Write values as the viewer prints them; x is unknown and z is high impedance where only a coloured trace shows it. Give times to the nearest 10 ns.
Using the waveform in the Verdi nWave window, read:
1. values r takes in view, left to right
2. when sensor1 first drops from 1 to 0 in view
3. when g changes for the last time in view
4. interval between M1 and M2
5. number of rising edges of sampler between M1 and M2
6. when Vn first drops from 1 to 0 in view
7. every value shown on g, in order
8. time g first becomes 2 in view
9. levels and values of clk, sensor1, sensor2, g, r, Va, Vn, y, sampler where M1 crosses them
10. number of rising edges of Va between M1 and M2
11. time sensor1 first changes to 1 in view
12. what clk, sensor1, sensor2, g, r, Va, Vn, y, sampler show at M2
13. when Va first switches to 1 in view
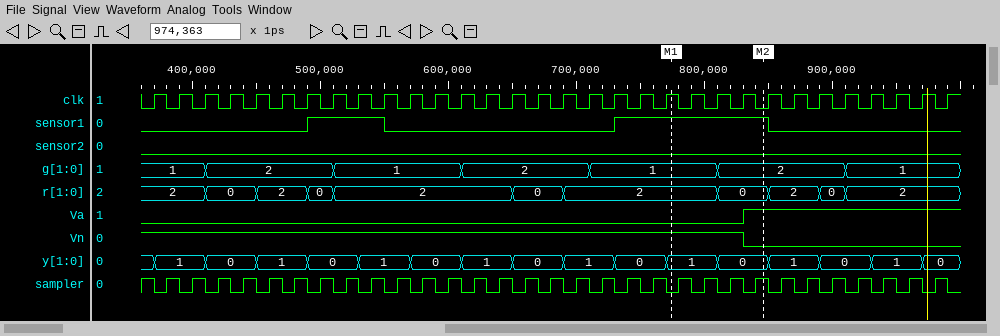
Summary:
2, 0, 2, 0, 2, 0, 2, 0, 2, 0, 2
550 ns
910 ns
70 ns
4
830 ns
1, 2, 1, 2, 1, 2, 1
410 ns
clk=1, sensor1=1, sensor2=0, g=1, r=2, Va=0, Vn=1, y=1, sampler=0
1
490 ns
clk=0, sensor1=1, sensor2=0, g=2, r=0, Va=1, Vn=0, y=0, sampler=1
830 ns
